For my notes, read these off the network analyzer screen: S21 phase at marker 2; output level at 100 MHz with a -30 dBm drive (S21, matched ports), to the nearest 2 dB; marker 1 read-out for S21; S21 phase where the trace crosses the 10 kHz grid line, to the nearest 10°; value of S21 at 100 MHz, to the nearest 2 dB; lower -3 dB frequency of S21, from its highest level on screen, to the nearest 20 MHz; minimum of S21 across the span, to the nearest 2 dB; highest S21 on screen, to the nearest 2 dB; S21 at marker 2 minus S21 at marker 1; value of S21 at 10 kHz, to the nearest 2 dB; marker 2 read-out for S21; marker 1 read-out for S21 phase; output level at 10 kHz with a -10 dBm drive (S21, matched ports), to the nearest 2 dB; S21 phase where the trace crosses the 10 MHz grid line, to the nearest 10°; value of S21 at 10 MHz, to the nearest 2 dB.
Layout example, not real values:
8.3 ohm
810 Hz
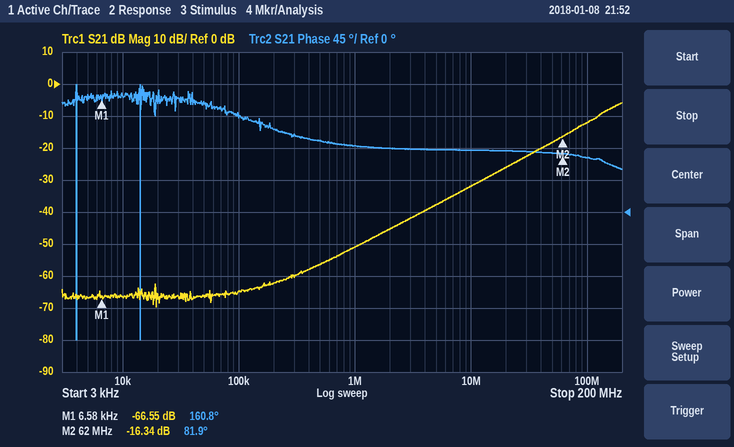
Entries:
81.9°
-42 dBm
-66.55 dB
160°
-12 dB
140 MHz
-70 dB
-6 dB
50.21 dB
-66 dB
-16.34 dB
160.8°
-76 dBm
90°
-32 dB
